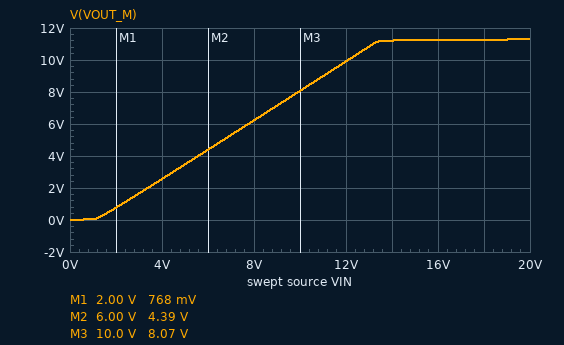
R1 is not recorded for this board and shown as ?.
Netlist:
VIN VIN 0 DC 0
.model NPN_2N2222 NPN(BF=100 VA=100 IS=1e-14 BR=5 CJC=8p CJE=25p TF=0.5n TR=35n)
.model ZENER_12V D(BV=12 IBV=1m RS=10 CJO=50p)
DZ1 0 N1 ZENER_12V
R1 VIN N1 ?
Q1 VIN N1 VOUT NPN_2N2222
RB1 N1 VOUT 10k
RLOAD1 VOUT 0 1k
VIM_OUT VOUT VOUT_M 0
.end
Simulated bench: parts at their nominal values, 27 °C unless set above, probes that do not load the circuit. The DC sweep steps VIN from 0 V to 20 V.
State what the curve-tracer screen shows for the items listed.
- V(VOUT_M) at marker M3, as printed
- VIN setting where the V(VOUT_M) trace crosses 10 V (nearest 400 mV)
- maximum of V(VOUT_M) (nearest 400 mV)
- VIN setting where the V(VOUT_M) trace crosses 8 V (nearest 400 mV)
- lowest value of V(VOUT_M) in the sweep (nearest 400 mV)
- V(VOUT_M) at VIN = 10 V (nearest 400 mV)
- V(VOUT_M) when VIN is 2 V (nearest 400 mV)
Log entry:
8.07 V
12.0 V
11.2 V
10.0 V
0 V
8.0 V
800 mV
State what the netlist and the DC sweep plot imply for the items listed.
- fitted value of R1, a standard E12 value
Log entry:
8.2 kΩ
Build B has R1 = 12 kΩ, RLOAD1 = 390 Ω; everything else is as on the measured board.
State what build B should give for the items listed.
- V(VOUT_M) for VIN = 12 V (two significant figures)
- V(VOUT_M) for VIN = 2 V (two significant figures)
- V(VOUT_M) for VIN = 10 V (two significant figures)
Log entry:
8.0 V
430 mV
6.5 V
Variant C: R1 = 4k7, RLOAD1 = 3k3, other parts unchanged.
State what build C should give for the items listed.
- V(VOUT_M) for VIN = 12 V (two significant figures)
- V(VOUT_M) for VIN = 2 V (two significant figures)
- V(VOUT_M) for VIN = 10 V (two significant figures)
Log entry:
11 V
1.1 V
8.9 V
